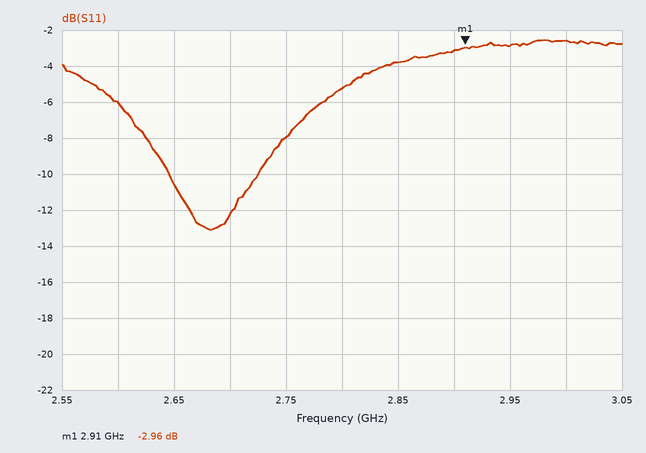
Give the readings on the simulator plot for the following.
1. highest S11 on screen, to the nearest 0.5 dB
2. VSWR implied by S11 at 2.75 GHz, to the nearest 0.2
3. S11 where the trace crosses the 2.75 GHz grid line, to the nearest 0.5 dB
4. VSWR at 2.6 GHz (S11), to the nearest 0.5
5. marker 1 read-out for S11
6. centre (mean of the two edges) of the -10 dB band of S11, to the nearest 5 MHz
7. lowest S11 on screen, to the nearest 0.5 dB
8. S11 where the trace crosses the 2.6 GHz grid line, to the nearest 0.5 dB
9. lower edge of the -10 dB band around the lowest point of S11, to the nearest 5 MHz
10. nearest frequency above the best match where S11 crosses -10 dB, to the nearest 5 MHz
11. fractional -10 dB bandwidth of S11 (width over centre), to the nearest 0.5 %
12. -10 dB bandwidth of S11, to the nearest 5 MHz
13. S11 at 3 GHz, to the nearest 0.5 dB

-2.5 dB
2.4
-8.0 dB
3.0
-2.96 dB
2.685 GHz
-13.0 dB
-6.0 dB
2.645 GHz
2.725 GHz
3.0 %
80 MHz
-2.5 dB
